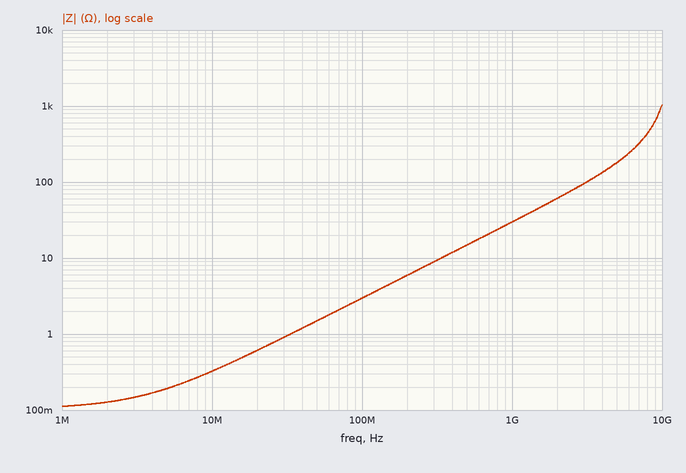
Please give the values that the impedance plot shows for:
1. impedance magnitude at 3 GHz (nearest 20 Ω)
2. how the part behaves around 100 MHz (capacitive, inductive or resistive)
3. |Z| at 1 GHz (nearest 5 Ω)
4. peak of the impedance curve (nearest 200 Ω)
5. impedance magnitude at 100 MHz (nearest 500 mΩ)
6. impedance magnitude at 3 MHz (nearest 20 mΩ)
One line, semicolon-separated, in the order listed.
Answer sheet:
100 Ω; inductive; 30 Ω; 1.0 kΩ; 3.0 Ω; 140 mΩ
